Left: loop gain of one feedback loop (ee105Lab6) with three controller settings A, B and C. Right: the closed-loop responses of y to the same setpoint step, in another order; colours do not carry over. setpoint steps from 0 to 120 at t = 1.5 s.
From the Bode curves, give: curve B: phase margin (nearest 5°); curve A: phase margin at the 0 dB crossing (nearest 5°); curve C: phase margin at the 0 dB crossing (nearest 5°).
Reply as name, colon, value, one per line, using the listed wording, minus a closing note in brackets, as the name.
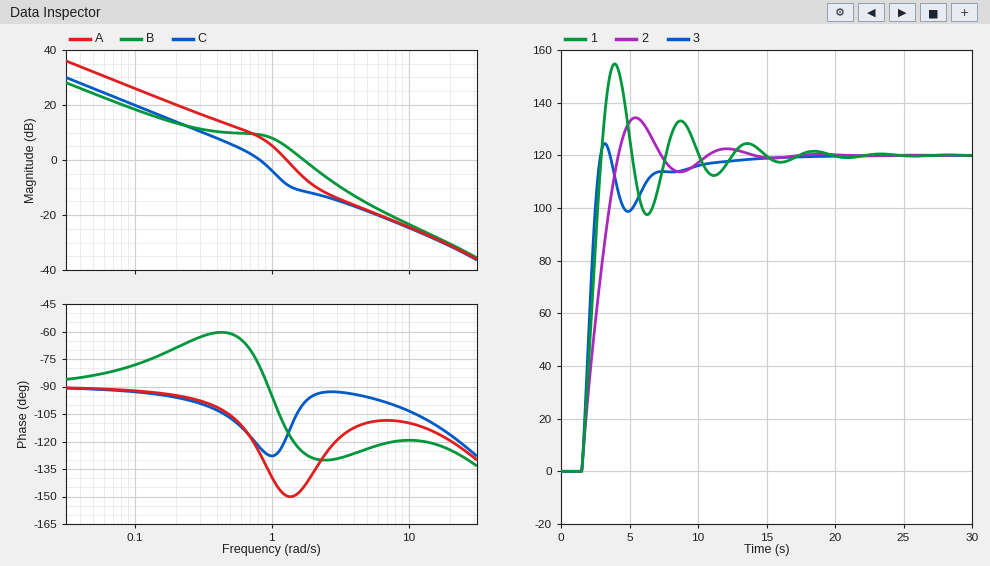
curve B: phase margin: 55°
curve A: phase margin at the 0 dB crossing: 30°
curve C: phase margin at the 0 dB crossing: 55°
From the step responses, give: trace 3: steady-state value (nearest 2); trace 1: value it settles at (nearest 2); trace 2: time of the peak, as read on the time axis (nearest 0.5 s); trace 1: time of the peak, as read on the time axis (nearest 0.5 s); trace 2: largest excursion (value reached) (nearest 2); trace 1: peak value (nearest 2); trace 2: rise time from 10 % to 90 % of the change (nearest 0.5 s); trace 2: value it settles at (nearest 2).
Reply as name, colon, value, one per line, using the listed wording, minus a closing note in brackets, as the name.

trace 3: steady-state value: 120
trace 1: value it settles at: 120
trace 2: time of the peak, as read on the time axis: 5.5 s
trace 1: time of the peak, as read on the time axis: 4.0 s
trace 2: largest excursion (value reached): 134
trace 1: peak value: 154
trace 2: rise time from 10 % to 90 % of the change: 2.0 s
trace 2: value it settles at: 120
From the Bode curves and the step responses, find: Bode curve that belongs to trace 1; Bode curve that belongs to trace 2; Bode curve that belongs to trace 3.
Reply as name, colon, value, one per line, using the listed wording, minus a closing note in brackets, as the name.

Bode curve that belongs to trace 1: A
Bode curve that belongs to trace 2: C
Bode curve that belongs to trace 3: B
